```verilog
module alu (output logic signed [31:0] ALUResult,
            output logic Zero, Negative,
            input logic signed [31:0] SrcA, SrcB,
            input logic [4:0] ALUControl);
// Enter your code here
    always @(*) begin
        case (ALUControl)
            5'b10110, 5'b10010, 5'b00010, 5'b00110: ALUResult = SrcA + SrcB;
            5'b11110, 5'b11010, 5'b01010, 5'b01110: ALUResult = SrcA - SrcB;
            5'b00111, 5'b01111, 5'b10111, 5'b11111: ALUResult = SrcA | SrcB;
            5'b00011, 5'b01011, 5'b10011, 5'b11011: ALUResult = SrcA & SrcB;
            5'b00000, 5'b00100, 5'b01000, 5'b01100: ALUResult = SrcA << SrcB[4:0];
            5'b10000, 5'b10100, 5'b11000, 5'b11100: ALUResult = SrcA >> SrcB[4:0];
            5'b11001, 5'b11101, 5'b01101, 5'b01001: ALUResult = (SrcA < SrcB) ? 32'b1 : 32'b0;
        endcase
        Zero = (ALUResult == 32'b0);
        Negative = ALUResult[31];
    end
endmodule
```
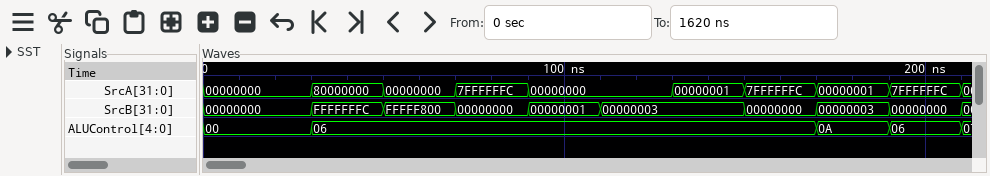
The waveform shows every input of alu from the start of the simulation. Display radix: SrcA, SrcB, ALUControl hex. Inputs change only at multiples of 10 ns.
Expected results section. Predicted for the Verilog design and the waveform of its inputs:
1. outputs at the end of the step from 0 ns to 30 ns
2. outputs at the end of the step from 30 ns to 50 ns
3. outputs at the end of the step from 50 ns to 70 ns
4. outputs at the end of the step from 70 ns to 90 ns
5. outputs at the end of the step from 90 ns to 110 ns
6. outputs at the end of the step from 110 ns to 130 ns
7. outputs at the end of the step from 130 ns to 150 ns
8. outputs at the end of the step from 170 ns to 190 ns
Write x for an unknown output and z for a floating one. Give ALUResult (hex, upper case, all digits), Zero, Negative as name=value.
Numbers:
ALUResult=00000000, Zero=1, Negative=0
ALUResult=7FFFFFFC, Zero=0, Negative=0
ALUResult=FFFFF800, Zero=0, Negative=1
ALUResult=7FFFFFFC, Zero=0, Negative=0
ALUResult=00000001, Zero=0, Negative=0
ALUResult=00000003, Zero=0, Negative=0
ALUResult=00000004, Zero=0, Negative=0
ALUResult=FFFFFFFE, Zero=0, Negative=1
